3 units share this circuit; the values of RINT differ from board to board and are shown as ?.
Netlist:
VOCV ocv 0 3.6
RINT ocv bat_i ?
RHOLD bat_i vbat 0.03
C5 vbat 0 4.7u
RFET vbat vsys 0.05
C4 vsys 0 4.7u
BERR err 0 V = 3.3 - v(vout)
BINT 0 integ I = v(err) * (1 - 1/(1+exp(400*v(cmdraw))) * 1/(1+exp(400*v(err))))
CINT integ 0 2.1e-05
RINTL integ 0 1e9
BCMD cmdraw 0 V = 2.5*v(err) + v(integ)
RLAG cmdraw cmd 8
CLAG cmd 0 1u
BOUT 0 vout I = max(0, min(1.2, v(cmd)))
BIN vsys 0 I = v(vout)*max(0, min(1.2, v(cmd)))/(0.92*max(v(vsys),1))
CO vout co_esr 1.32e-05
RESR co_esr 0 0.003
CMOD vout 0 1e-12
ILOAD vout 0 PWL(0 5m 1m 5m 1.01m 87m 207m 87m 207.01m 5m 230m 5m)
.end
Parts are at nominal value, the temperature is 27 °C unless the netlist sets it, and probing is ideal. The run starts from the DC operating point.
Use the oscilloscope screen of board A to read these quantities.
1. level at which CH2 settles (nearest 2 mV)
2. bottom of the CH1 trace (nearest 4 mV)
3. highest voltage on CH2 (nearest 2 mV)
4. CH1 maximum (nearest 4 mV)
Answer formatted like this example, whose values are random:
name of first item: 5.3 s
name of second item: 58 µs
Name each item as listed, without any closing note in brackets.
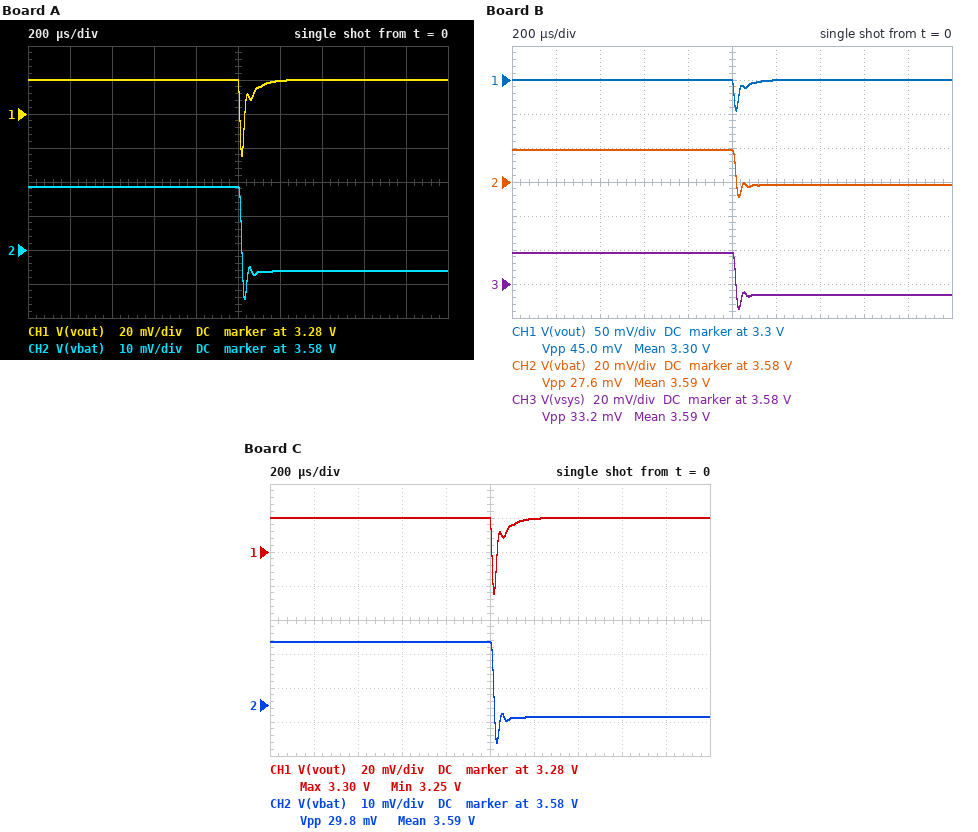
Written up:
level at which CH2 settles: 3.574 V
bottom of the CH1 trace: 3.256 V
highest voltage on CH2: 3.598 V
CH1 maximum: 3.300 V
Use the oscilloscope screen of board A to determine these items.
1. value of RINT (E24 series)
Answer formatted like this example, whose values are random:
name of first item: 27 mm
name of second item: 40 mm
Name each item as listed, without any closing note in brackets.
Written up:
value of RINT: 0.27 Ω
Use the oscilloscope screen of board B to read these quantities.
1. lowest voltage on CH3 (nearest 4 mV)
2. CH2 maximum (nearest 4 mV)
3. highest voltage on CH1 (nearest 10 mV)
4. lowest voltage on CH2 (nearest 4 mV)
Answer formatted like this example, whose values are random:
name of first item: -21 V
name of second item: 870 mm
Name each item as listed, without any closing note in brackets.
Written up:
lowest voltage on CH3: 3.564 V
CH2 maximum: 3.600 V
highest voltage on CH1: 3.30 V
lowest voltage on CH2: 3.572 V
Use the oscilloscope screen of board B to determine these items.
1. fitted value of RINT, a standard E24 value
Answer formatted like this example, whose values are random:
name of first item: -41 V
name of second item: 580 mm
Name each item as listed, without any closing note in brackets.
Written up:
fitted value of RINT, a standard E24 value: 0.22 Ω
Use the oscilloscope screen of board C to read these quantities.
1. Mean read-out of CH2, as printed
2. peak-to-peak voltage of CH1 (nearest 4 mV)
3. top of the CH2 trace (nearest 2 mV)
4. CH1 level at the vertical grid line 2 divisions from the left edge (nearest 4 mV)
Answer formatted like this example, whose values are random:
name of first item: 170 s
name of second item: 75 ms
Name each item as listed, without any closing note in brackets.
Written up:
Mean read-out of CH2, as printed: 3.59 V
peak-to-peak voltage of CH1: 44 mV
top of the CH2 trace: 3.598 V
CH1 level at the vertical grid line 2 divisions from the left edge: 3.300 V
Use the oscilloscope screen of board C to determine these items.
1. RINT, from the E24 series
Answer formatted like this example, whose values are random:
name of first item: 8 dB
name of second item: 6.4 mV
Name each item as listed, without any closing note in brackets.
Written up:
RINT, from the E24 series: 0.24 Ω
